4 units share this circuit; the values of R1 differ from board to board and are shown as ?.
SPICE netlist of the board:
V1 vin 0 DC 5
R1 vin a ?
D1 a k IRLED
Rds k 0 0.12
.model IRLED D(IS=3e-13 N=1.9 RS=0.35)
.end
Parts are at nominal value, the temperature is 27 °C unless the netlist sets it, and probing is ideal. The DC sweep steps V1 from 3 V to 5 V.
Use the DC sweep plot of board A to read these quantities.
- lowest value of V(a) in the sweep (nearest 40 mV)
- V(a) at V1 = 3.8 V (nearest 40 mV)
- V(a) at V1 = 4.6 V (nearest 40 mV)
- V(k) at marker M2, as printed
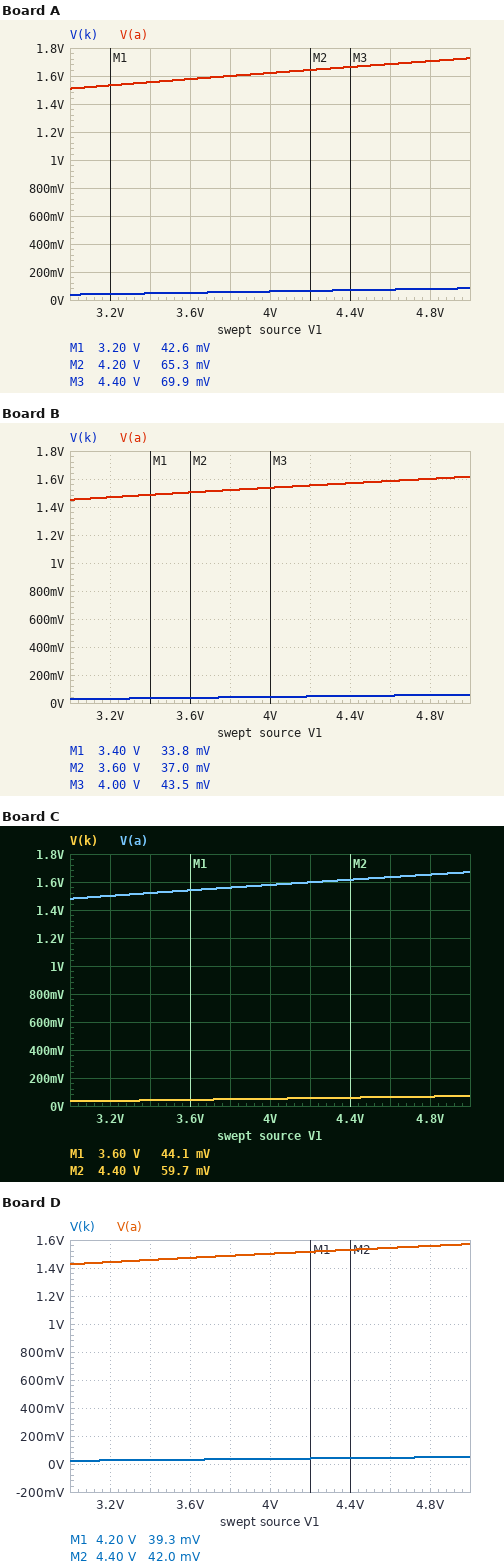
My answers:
1.52 V
1.60 V
1.68 V
65.3 mV
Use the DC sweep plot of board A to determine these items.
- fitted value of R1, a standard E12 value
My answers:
4.7 Ω
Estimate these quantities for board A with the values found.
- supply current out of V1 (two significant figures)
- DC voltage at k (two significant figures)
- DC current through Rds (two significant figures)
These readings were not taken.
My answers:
700 mA
84 mV
700 mA
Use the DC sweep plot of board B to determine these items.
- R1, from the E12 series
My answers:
6.8 Ω
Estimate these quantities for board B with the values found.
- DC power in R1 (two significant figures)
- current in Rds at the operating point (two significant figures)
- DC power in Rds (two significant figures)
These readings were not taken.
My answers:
1.7 W
500 mA
30 mW
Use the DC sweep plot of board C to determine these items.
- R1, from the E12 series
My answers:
5.6 Ω
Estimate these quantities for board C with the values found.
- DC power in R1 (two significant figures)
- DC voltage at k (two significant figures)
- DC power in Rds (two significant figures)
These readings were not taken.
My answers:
2.0 W
71 mV
42 mW
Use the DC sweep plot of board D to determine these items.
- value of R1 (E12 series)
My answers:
8.2 Ω
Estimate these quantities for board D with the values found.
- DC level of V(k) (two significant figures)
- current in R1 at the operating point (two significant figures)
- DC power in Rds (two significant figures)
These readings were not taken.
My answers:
50 mV
420 mA
21 mW
